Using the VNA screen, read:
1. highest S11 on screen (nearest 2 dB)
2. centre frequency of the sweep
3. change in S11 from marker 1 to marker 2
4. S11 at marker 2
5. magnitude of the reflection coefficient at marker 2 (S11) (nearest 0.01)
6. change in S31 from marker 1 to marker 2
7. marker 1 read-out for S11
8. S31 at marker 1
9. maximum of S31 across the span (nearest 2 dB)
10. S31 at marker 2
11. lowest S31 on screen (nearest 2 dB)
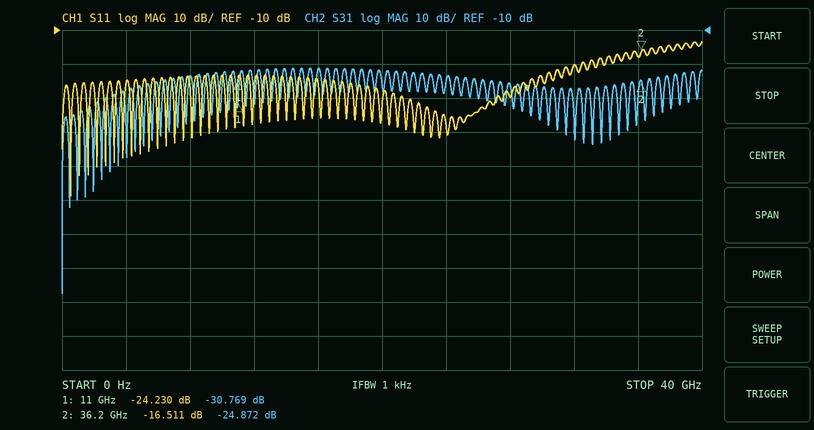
-14 dB
20 GHz
7.719 dB
-16.511 dB
0.15
5.897 dB
-24.230 dB
-30.769 dB
-22 dB
-24.872 dB
-88 dB
